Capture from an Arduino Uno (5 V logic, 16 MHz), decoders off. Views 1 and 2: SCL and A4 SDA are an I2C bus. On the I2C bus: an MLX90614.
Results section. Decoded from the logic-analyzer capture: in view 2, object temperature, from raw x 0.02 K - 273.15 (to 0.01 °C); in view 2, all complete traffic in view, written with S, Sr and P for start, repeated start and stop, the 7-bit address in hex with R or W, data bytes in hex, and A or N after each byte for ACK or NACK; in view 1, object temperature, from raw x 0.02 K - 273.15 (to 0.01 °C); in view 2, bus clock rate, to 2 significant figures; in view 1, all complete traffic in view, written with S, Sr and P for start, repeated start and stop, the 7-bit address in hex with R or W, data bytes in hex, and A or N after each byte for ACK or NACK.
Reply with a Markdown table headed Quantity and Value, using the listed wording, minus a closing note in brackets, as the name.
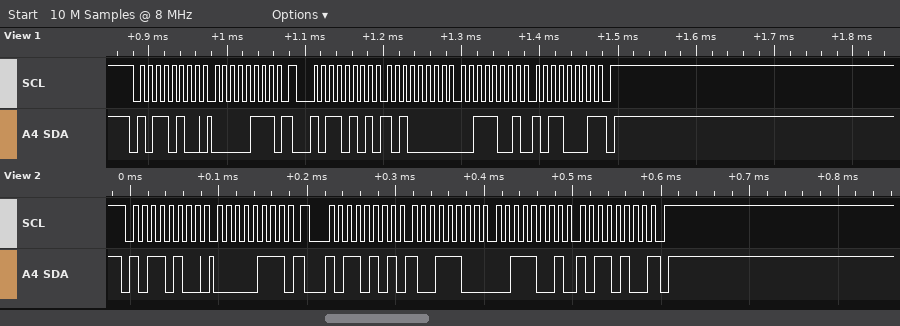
| Quantity | Value |
|---|---|
| in view 2, object temperature, from raw x 0.02 K - 273.15 | 21.81 °C |
| in view 2, all complete traffic in view, written with S, Sr and P for start, repeated start and stop, the 7-bit address in hex with R or W, data bytes in hex, and A or N after each byte for ACK or NACK | S 5AW A 07 A Sr 5AR A 9C A 39 A B4 N P |
| in view 1, object temperature, from raw x 0.02 K - 273.15 | 21.89 °C |
| in view 2, bus clock rate, to 2 significant figures | 100 kHz |
| in view 1, all complete traffic in view, written with S, Sr and P for start, repeated start and stop, the 7-bit address in hex with R or W, data bytes in hex, and A or N after each byte for ACK or NACK | S 5AW A 07 A Sr 5AR A A0 A 39 A B1 N P |
